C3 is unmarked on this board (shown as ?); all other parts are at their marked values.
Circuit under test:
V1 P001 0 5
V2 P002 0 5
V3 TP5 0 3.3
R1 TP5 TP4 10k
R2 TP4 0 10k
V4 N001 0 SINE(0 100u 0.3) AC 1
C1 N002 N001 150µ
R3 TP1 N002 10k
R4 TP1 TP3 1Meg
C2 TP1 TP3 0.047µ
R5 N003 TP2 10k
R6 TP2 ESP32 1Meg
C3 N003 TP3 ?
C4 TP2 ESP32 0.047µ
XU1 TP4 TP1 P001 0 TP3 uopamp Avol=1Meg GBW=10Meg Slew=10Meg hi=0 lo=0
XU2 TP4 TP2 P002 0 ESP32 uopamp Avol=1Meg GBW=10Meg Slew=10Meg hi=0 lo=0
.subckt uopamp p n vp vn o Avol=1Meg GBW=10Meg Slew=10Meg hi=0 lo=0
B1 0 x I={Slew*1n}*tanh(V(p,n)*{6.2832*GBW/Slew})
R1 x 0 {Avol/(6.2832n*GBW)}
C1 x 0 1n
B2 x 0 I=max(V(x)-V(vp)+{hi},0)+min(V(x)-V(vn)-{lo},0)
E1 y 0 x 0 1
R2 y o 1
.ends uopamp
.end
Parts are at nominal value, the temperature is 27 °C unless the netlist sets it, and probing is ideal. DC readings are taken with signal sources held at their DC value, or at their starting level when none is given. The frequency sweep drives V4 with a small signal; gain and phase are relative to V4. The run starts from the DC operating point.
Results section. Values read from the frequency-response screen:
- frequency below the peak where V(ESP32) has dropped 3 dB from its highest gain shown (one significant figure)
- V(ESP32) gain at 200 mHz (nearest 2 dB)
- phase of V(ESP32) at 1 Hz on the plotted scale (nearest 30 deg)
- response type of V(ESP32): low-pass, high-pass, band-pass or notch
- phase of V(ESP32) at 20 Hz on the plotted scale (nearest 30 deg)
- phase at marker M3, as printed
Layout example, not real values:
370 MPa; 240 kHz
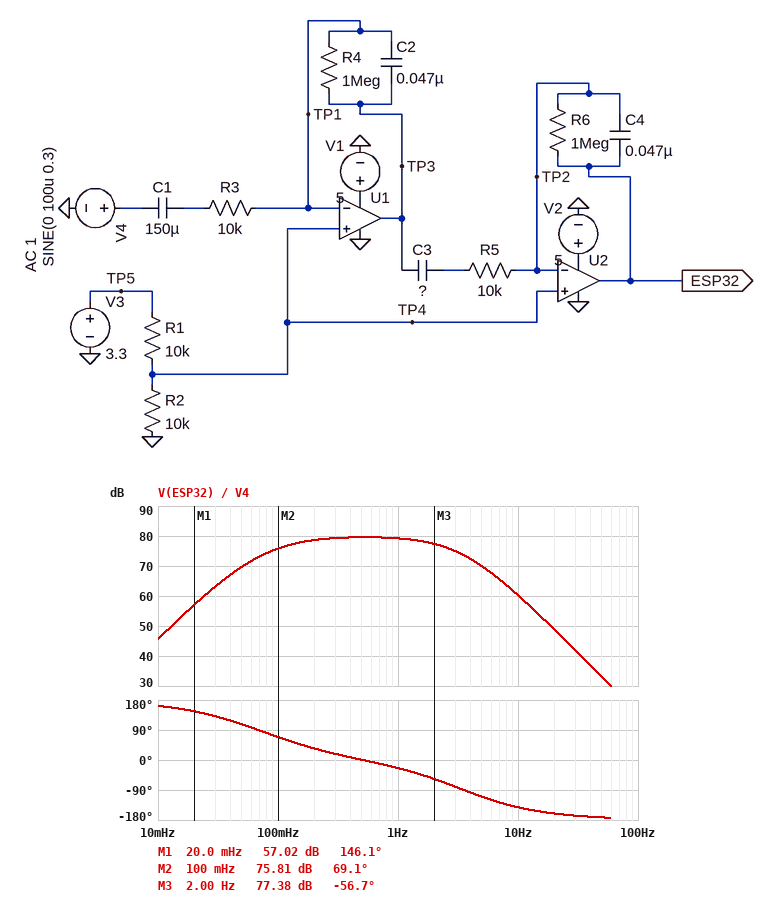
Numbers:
100 mHz; 78 dB; -30 deg; band-pass; -150 deg; -56.7 deg
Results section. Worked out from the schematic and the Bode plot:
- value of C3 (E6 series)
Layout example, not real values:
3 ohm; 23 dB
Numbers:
330 µF
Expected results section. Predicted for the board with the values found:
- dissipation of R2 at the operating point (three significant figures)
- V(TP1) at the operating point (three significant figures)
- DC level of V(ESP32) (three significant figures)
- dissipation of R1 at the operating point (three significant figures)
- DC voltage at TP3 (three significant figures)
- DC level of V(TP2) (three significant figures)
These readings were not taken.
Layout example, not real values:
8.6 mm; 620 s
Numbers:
272 µW; 1.65 V; 1.65 V; 272 µW; 1.65 V; 1.65 V
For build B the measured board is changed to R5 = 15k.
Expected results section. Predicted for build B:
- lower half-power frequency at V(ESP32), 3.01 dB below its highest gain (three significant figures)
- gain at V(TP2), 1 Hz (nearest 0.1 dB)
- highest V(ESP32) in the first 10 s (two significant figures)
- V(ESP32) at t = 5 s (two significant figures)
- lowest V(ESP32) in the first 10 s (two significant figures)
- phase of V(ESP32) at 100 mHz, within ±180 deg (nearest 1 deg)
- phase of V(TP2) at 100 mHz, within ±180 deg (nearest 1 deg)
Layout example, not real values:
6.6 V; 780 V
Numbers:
106 mHz; -44.3 dB; 2.3 V; 1.5 V; 980 mV; 61 deg; -118 deg
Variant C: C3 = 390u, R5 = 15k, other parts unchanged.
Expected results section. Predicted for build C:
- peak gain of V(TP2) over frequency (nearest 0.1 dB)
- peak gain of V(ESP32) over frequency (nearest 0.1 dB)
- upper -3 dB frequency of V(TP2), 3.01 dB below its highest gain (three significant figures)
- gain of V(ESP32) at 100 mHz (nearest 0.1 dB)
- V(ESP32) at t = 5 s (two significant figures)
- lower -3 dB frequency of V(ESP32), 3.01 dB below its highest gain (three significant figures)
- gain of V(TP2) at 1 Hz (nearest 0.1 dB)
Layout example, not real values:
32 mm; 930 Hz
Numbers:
-43.9 dB; 76.1 dB; 2.44 Hz; 72.9 dB; 1.5 V; 104 mHz; -44.3 dB
